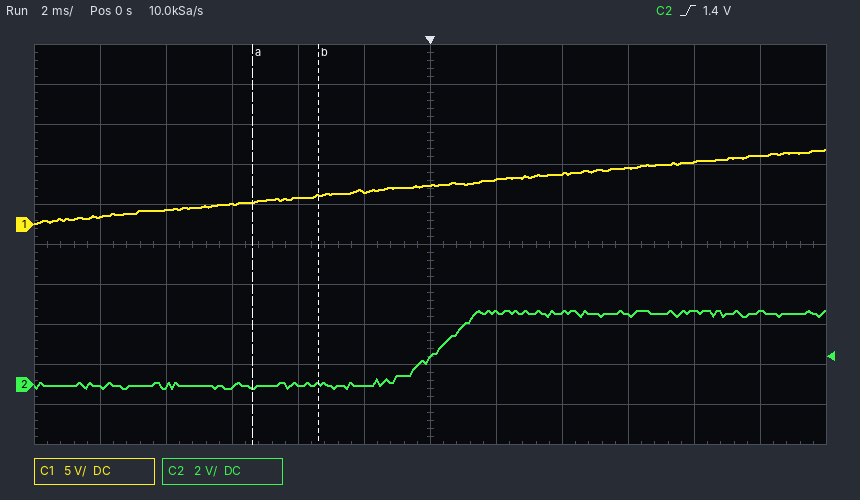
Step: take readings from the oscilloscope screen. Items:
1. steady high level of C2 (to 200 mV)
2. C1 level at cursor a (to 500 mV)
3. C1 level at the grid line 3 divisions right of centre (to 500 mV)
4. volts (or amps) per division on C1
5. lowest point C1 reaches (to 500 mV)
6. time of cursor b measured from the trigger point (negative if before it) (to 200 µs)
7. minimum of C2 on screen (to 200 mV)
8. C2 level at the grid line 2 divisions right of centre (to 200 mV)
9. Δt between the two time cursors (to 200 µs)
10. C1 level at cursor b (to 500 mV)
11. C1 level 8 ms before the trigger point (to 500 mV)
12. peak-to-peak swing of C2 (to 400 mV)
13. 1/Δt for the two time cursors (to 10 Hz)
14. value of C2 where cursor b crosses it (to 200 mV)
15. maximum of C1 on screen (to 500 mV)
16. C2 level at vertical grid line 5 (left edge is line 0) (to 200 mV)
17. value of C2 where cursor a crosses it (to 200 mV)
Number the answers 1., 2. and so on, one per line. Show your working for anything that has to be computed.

1. 3.6 V
2. 3.0 V
3. 7.0 V
4. 5 V
5. 0.0 V
6. -3.4 ms
7. -200 mV
8. 3.6 V
9. 2.0 ms
10. 3.5 V
11. 2.0 V
12. 4.0 V
13. 1 / 2.0 ms ≈ 500 Hz
14. 0.0 V
15. 9.5 V
16. 0.0 V
17. -200 mV
